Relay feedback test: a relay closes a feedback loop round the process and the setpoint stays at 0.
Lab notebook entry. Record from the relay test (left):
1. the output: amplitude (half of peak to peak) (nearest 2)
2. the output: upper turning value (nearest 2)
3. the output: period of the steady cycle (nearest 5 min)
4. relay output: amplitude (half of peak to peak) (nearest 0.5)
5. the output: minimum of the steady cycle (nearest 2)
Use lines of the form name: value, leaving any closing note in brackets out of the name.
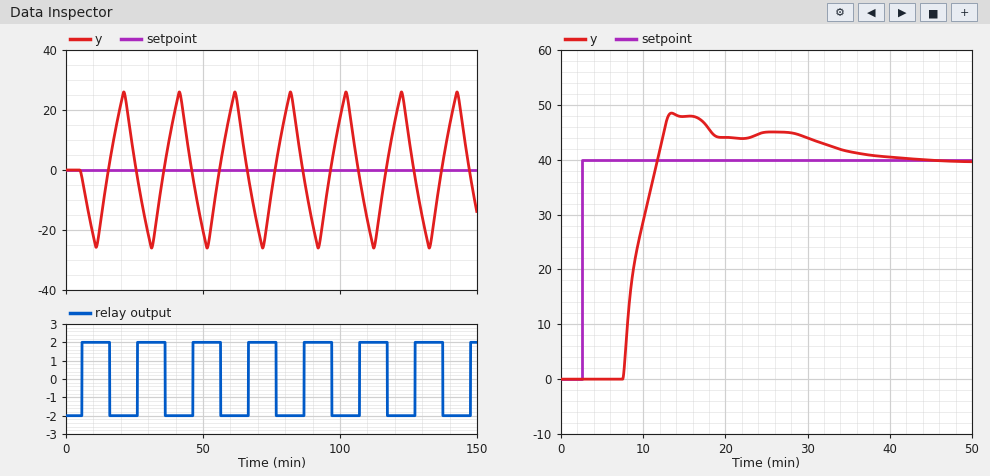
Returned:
the output: amplitude (half of peak to peak): 26
the output: upper turning value: 26
the output: period of the steady cycle: 20 min
relay output: amplitude (half of peak to peak): 2.0
the output: minimum of the steady cycle: -26
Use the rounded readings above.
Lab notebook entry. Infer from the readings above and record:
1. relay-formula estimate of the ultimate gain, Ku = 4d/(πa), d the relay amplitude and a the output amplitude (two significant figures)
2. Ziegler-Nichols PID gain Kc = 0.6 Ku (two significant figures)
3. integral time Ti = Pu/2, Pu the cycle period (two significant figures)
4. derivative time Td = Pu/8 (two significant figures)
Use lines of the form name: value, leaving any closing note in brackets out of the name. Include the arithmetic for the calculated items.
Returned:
relay-formula estimate of the ultimate gain, Ku = 4d/(πa), d the relay amplitude and a the output amplitude: 4 × 2 / (π × 26) = 0.098
Ziegler-Nichols PID gain Kc = 0.6 Ku: 0.6 × 0.098 = 0.059
integral time Ti = Pu/2, Pu the cycle period: 20 / 2 = 10 min
derivative time Td = Pu/8: 20 / 8 = 2.5 min
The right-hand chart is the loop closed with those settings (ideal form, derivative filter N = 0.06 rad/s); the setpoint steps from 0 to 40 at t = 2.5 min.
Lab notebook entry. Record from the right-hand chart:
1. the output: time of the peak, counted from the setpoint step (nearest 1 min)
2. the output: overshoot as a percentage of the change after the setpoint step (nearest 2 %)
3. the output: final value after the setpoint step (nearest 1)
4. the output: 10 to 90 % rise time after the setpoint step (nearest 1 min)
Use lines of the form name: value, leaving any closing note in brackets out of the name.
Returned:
the output: time of the peak, counted from the setpoint step: 11 min
the output: overshoot as a percentage of the change after the setpoint step: 22 %
the output: final value after the setpoint step: 40
the output: 10 to 90 % rise time after the setpoint step: 3 min
